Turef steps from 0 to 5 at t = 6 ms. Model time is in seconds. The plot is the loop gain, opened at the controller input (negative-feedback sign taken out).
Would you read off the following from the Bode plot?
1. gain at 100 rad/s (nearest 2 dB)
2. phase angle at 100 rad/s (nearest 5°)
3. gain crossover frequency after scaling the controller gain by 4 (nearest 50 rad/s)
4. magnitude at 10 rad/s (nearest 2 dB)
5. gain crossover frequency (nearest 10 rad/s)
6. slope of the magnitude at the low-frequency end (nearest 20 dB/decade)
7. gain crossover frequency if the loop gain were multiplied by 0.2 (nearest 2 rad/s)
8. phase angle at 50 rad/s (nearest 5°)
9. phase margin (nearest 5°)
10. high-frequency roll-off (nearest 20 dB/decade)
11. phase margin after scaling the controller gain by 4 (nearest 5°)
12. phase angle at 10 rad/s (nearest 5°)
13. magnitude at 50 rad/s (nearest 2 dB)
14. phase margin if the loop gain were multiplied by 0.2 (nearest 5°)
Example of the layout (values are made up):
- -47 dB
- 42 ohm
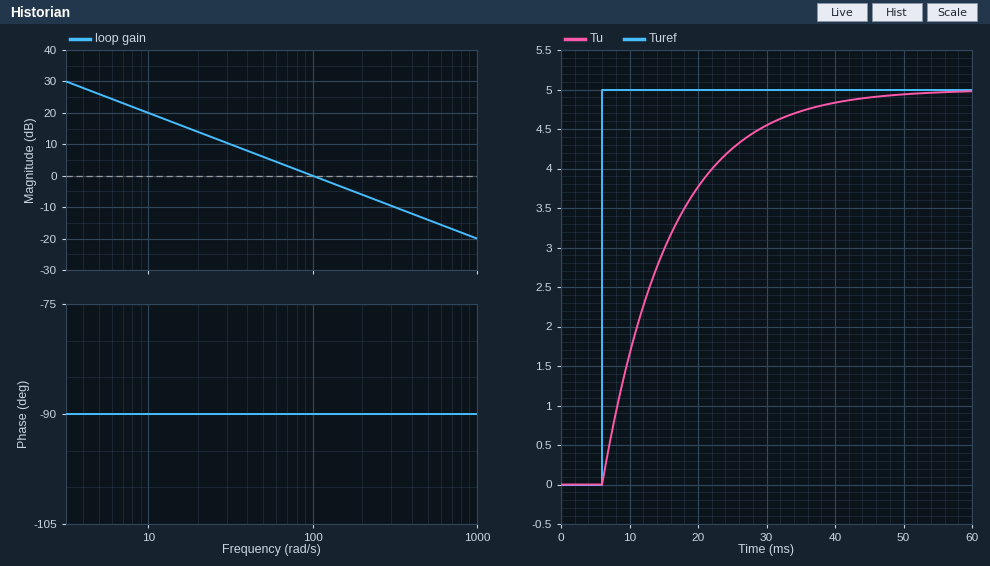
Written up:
- 0 dB
- -90°
- 400 rad/s
- 20 dB
- 100 rad/s
- -20 dB/decade
- 20 rad/s
- -90°
- 90°
- -20 dB/decade
- 90°
- -90°
- 6 dB
- 90°
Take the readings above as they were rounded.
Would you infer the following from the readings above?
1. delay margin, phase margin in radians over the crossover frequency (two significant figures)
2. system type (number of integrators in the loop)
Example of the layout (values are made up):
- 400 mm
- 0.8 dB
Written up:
- 0.016 s
- 1
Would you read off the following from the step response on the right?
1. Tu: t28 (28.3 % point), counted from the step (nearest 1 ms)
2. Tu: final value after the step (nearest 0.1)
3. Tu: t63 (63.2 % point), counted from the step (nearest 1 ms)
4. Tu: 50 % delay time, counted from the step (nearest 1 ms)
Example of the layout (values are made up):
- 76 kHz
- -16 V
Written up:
- 3 ms
- 5.0
- 10 ms
- 7 ms
